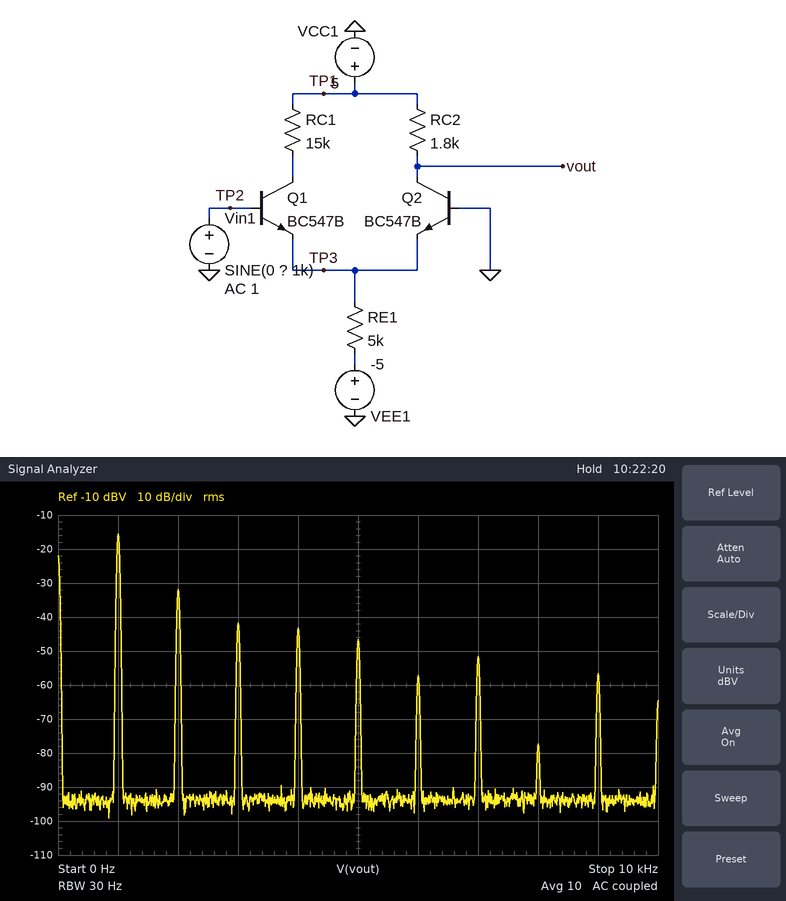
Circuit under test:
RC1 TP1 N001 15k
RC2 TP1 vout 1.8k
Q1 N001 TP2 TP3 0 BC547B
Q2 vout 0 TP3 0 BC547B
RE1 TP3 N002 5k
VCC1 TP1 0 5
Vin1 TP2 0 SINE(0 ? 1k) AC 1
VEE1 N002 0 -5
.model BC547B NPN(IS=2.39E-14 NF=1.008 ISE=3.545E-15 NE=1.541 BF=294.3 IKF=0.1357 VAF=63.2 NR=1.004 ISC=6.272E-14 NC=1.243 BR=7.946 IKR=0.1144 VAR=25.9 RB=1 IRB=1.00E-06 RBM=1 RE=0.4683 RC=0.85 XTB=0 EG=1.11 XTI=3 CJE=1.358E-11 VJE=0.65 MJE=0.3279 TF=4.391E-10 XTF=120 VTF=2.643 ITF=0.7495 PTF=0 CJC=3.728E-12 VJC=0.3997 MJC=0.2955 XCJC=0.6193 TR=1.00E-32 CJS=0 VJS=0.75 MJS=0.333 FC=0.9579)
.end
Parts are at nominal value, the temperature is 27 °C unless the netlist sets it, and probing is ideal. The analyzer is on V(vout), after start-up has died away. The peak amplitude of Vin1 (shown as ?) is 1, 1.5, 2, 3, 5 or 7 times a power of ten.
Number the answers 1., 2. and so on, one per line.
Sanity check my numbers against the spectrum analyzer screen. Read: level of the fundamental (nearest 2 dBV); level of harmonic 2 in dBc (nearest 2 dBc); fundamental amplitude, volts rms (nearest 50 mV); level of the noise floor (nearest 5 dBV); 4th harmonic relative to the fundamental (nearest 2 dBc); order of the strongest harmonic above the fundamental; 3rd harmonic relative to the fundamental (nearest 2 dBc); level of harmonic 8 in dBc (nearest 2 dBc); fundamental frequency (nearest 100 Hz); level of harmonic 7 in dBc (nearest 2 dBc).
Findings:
1. -16 dBV
2. -16 dBc
3. 150 mV
4. -95 dBV
5. -28 dBc
6. 2
7. -26 dBc
8. -62 dBc
9. 1.0 kHz
10. -36 dBc
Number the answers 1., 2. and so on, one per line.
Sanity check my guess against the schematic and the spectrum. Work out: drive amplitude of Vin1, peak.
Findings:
1. 30 mV
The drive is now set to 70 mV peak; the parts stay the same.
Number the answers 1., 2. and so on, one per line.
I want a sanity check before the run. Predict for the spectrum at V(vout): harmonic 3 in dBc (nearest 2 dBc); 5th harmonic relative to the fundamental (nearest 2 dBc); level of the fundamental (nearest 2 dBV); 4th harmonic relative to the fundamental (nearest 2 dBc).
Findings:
1. -42 dBc
2. -36 dBc
3. -8 dBV
4. -26 dBc
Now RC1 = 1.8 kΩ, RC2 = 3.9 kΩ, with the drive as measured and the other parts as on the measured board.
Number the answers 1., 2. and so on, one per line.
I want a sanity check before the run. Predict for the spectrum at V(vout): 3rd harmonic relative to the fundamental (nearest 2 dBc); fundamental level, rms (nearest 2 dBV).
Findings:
1. -32 dBc
2. -4 dBV
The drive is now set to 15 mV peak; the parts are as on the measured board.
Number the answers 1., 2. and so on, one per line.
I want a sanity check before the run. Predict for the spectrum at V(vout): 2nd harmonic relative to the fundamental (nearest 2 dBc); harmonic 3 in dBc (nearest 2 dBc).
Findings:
1. -14 dBc
2. -20 dBc
